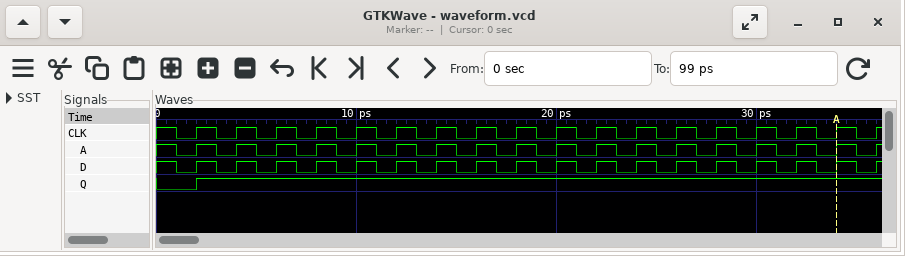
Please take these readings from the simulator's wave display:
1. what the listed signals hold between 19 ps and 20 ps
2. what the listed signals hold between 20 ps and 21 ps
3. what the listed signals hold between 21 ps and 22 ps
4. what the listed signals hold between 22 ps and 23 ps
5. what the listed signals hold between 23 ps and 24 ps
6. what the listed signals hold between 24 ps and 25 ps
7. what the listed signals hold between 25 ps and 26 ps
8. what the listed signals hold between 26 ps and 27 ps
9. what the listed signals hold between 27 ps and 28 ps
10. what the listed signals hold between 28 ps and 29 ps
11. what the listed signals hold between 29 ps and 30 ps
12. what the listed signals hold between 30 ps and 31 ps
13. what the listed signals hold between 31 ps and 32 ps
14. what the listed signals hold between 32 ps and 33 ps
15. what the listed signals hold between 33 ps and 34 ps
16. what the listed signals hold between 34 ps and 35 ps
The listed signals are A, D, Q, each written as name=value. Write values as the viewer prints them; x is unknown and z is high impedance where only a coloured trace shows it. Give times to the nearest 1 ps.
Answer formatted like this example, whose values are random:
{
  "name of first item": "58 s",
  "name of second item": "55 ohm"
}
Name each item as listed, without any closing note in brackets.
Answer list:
{
  "what the listed signals hold between 19 ps and 20 ps": "A=0, D=0, Q=1",
  "what the listed signals hold between 20 ps and 21 ps": "A=1, D=1, Q=1",
  "what the listed signals hold between 21 ps and 22 ps": "A=0, D=0, Q=1",
  "what the listed signals hold between 22 ps and 23 ps": "A=1, D=1, Q=1",
  "what the listed signals hold between 23 ps and 24 ps": "A=0, D=0, Q=1",
  "what the listed signals hold between 24 ps and 25 ps": "A=1, D=1, Q=1",
  "what the listed signals hold between 25 ps and 26 ps": "A=0, D=0, Q=1",
  "what the listed signals hold between 26 ps and 27 ps": "A=1, D=1, Q=1",
  "what the listed signals hold between 27 ps and 28 ps": "A=0, D=0, Q=1",
  "what the listed signals hold between 28 ps and 29 ps": "A=1, D=1, Q=1",
  "what the listed signals hold between 29 ps and 30 ps": "A=0, D=0, Q=1",
  "what the listed signals hold between 30 ps and 31 ps": "A=1, D=1, Q=1",
  "what the listed signals hold between 31 ps and 32 ps": "A=0, D=0, Q=1",
  "what the listed signals hold between 32 ps and 33 ps": "A=1, D=1, Q=1",
  "what the listed signals hold between 33 ps and 34 ps": "A=0, D=0, Q=1",
  "what the listed signals hold between 34 ps and 35 ps": "A=1, D=1, Q=1"
}
